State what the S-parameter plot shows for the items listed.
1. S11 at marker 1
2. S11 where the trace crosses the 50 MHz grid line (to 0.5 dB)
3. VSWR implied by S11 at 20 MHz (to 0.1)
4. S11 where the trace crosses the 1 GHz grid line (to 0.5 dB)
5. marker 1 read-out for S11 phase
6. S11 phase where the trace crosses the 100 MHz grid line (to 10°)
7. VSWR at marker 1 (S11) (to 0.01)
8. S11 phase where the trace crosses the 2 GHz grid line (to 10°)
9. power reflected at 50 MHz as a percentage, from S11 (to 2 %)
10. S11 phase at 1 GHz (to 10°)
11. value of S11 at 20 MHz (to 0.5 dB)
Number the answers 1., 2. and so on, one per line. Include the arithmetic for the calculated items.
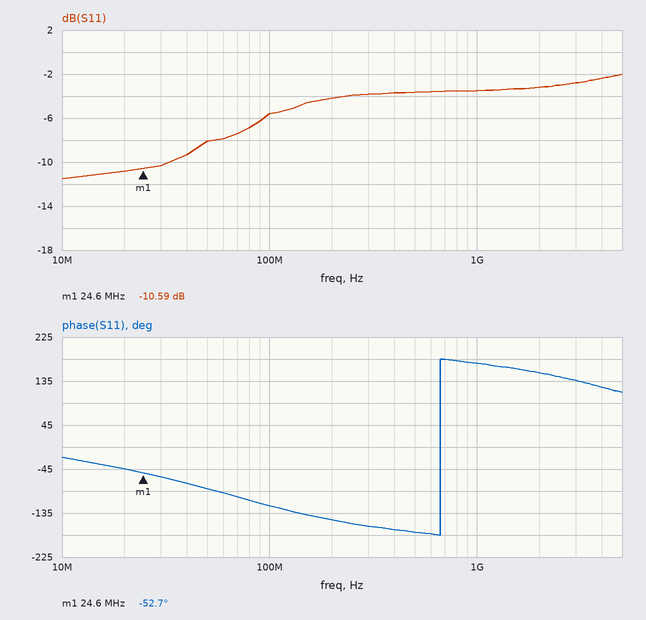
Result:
1. -10.59 dB
2. -8.0 dB
3. |Γ| = 10^(-11/20) = 0.2818; VSWR = (1 + 0.2818)/(1 − 0.2818) ≈ 1.8
4. -3.5 dB
5. -52.7°
6. -120°
7. (1 + 0.2955)/(1 − 0.2955) ≈ 1.84
8. 150°
9. 10^(-8/10) ≈ 16 %
10. 170°
11. -11.0 dB
